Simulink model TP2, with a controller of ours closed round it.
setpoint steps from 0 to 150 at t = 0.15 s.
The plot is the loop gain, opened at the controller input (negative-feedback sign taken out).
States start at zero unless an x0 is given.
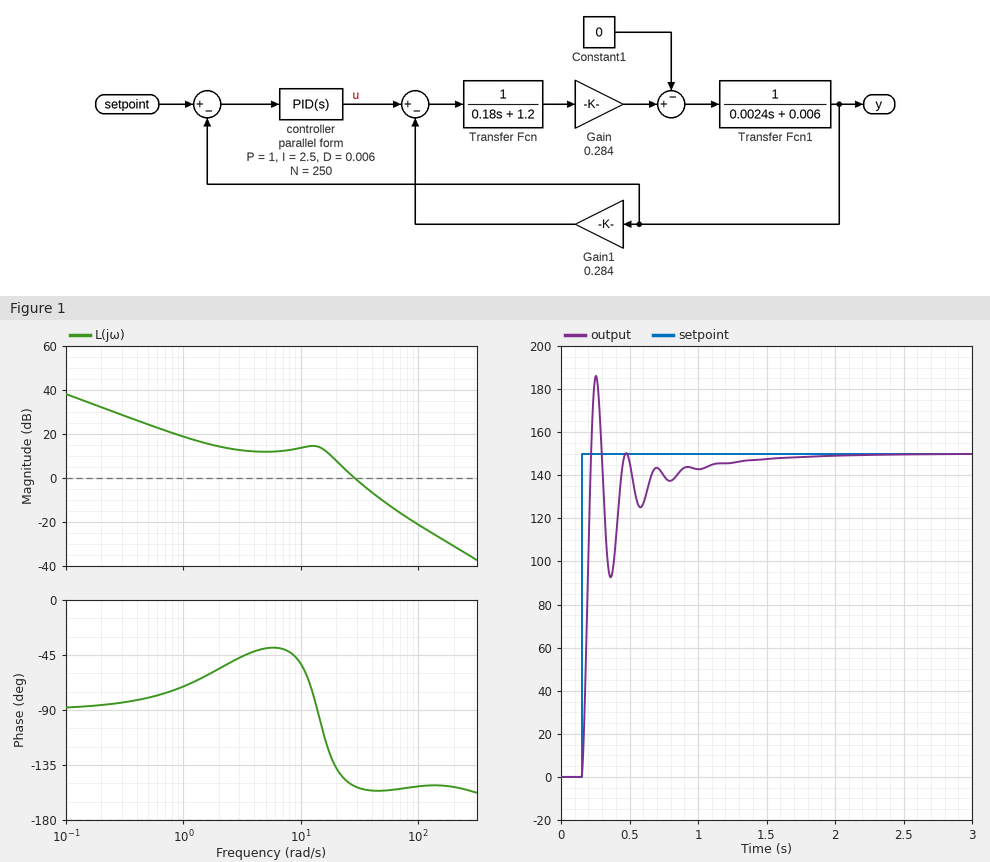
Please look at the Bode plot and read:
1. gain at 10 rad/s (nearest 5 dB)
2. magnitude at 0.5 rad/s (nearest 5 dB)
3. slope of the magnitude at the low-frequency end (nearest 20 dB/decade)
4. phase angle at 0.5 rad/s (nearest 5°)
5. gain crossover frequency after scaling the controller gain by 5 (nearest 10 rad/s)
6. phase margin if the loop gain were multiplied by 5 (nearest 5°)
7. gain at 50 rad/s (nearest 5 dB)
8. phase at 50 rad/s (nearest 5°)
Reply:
15 dB
25 dB
-20 dB/decade
-80°
60 rad/s
25°
-10 dB
-155°
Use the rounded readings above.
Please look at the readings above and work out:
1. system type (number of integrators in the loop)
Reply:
1
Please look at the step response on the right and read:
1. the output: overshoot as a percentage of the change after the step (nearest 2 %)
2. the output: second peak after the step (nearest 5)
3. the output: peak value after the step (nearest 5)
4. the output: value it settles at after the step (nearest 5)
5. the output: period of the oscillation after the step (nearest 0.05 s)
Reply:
24 %
150
185
150
0.20 s
